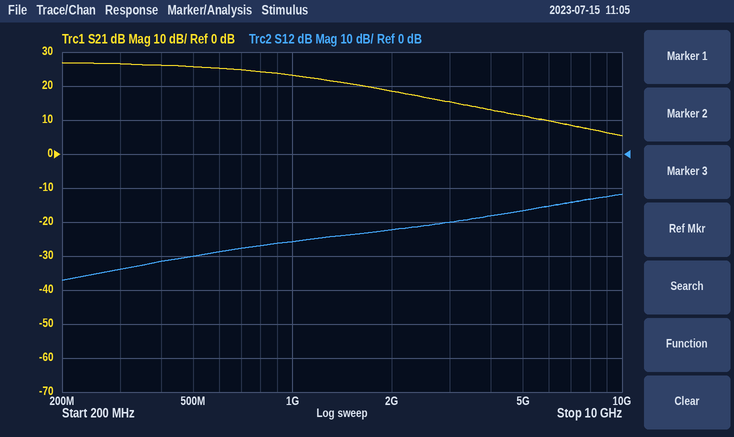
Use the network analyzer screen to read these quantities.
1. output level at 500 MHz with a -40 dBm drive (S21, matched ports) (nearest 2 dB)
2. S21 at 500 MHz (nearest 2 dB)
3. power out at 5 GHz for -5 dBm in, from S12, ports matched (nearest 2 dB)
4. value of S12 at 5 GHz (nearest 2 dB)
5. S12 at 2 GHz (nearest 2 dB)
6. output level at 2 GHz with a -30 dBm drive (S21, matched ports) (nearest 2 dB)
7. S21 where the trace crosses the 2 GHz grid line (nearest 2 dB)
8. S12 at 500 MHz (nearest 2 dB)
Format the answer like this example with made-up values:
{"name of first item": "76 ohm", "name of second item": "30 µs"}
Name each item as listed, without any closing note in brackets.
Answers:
{"output level at 500 MHz with a -40 dBm drive (S21, matched ports)": "-14 dBm", "S21 at 500 MHz": "26 dB", "power out at 5 GHz for -5 dBm in, from S12, ports matched": "-22 dBm", "value of S12 at 5 GHz": "-16 dB", "S12 at 2 GHz": "-22 dB", "output level at 2 GHz with a -30 dBm drive (S21, matched ports)": "-12 dBm", "S21 where the trace crosses the 2 GHz grid line": "18 dB", "S12 at 500 MHz": "-30 dB"}
